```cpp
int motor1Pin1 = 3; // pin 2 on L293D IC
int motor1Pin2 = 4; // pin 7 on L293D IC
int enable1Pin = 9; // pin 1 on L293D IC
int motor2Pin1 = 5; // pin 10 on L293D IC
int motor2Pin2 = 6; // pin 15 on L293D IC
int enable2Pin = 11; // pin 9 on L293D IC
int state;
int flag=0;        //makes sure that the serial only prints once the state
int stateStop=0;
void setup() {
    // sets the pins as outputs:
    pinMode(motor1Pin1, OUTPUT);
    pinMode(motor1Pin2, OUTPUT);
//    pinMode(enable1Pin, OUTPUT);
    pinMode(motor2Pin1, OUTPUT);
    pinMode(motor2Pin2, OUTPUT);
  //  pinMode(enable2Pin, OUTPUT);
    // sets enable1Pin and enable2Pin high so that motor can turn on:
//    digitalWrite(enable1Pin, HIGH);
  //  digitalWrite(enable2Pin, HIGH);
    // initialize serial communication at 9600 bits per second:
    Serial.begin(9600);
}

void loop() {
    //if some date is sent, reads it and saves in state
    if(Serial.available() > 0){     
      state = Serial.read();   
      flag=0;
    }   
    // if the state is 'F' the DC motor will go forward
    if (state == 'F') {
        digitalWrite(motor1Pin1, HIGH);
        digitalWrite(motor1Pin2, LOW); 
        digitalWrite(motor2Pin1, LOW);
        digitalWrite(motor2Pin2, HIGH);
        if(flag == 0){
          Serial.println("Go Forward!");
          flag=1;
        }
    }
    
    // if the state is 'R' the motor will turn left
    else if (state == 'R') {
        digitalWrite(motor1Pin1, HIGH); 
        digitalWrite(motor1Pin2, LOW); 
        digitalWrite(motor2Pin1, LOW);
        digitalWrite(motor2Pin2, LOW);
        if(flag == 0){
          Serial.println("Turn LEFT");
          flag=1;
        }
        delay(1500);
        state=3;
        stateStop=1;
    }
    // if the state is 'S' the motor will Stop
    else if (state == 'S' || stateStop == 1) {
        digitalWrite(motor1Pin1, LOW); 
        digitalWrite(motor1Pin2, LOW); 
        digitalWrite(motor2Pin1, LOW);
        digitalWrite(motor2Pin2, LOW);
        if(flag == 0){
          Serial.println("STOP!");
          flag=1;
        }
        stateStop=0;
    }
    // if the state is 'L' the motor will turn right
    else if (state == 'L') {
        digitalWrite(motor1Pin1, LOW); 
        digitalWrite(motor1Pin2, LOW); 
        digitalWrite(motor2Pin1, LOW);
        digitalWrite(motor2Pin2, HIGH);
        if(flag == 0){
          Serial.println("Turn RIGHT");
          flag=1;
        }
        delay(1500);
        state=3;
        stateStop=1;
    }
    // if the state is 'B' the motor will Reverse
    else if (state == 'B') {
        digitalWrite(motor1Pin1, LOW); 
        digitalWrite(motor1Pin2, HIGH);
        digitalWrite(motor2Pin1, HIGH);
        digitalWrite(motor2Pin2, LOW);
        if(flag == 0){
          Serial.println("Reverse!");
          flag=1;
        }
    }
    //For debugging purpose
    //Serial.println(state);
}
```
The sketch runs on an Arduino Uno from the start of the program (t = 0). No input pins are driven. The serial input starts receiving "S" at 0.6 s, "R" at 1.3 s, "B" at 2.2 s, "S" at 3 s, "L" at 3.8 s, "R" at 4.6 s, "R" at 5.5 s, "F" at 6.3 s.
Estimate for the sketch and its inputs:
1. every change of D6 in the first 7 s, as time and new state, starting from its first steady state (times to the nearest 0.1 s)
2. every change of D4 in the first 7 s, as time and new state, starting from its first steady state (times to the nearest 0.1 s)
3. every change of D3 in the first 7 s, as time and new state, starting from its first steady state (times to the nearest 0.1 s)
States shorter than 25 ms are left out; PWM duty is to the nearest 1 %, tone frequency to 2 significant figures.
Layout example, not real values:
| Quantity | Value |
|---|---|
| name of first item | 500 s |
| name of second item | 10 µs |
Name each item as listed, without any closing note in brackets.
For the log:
| Quantity | Value |
|---|---|
| every change of D6 in the first 7 s, as time and new state, starting from its first steady state | 0 s low; 3.8 s high; 5.3 s low |
| every change of D4 in the first 7 s, as time and new state, starting from its first steady state | 0 s low; 2.8 s high; 3 s low |
| every change of D3 in the first 7 s, as time and new state, starting from its first steady state | 0 s low; 1.3 s high; 2.8 s low; 5.3 s high |
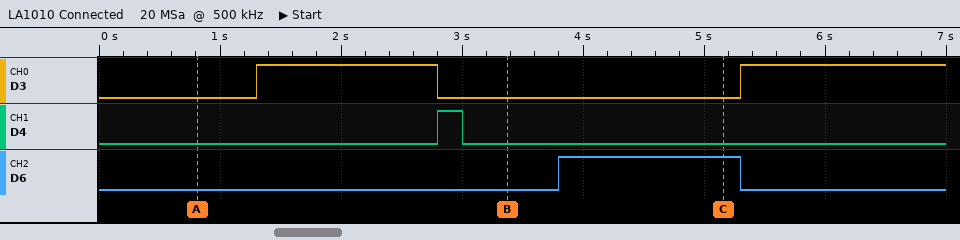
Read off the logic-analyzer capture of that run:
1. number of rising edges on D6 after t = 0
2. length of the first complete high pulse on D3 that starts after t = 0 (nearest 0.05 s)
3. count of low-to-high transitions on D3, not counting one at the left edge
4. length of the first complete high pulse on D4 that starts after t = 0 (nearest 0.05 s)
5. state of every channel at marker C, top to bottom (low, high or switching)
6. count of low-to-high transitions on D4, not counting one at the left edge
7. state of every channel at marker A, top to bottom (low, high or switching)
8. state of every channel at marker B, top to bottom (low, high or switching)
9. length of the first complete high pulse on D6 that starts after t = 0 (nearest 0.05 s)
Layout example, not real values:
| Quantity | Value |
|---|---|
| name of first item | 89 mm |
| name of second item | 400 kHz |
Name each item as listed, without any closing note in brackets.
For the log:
| Quantity | Value |
|---|---|
| number of rising edges on D6 after t = 0 | 1 |
| length of the first complete high pulse on D3 that starts after t = 0 | 1.50 s |
| count of low-to-high transitions on D3, not counting one at the left edge | 2 |
| length of the first complete high pulse on D4 that starts after t = 0 | 0.20 s |
| state of every channel at marker C, top to bottom | D3 low, D4 low, D6 high |
| count of low-to-high transitions on D4, not counting one at the left edge | 1 |
| state of every channel at marker A, top to bottom | D3 low, D4 low, D6 low |
| state of every channel at marker B, top to bottom | D3 low, D4 low, D6 low |
| length of the first complete high pulse on D6 that starts after t = 0 | 1.50 s |
